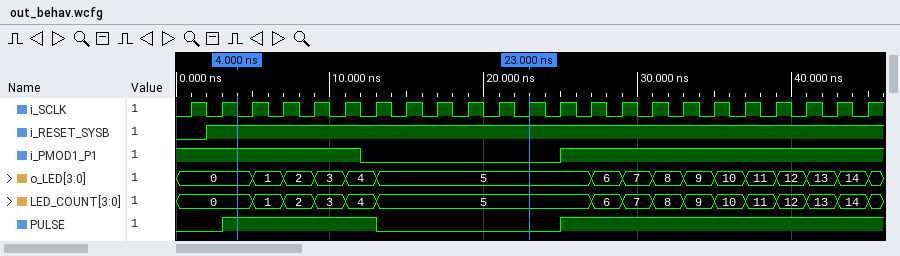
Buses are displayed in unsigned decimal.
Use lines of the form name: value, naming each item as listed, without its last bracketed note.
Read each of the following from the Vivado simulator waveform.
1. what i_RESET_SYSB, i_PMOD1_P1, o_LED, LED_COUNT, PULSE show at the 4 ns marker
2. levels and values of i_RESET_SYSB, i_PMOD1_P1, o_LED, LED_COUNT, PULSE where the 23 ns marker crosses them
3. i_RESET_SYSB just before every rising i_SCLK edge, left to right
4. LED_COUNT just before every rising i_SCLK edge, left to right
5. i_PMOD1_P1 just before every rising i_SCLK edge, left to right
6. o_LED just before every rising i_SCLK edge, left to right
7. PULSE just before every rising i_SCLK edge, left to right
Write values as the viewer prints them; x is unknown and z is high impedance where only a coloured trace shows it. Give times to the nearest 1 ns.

what i_RESET_SYSB, i_PMOD1_P1, o_LED, LED_COUNT, PULSE show at the 4 ns marker: i_RESET_SYSB=1, i_PMOD1_P1=1, o_LED=0, LED_COUNT=0, PULSE=1
levels and values of i_RESET_SYSB, i_PMOD1_P1, o_LED, LED_COUNT, PULSE where the 23 ns marker crosses them: i_RESET_SYSB=1, i_PMOD1_P1=0, o_LED=5, LED_COUNT=5, PULSE=0
i_RESET_SYSB just before every rising i_SCLK edge, left to right: 0 1 1 1 1 1 1 1 1 1 1 1 1 1 1 1 1 1 1 1 1 1 1
LED_COUNT just before every rising i_SCLK edge, left to right: 0, 0, 0, 1, 2, 3, 4, 5, 5, 5, 5, 5, 5, 5, 6, 7, 8, 9, 10, 11, 12, 13, 14
i_PMOD1_P1 just before every rising i_SCLK edge, left to right: 1 1 1 1 1 1 0 0 0 0 0 0 0 1 1 1 1 1 1 1 1 1 1
o_LED just before every rising i_SCLK edge, left to right: 0, 0, 0, 1, 2, 3, 4, 5, 5, 5, 5, 5, 5, 5, 6, 7, 8, 9, 10, 11, 12, 13, 14
PULSE just before every rising i_SCLK edge, left to right: 0 0 1 1 1 1 1 0 0 0 0 0 0 1 1 1 1 1 1 1 1 1 1
